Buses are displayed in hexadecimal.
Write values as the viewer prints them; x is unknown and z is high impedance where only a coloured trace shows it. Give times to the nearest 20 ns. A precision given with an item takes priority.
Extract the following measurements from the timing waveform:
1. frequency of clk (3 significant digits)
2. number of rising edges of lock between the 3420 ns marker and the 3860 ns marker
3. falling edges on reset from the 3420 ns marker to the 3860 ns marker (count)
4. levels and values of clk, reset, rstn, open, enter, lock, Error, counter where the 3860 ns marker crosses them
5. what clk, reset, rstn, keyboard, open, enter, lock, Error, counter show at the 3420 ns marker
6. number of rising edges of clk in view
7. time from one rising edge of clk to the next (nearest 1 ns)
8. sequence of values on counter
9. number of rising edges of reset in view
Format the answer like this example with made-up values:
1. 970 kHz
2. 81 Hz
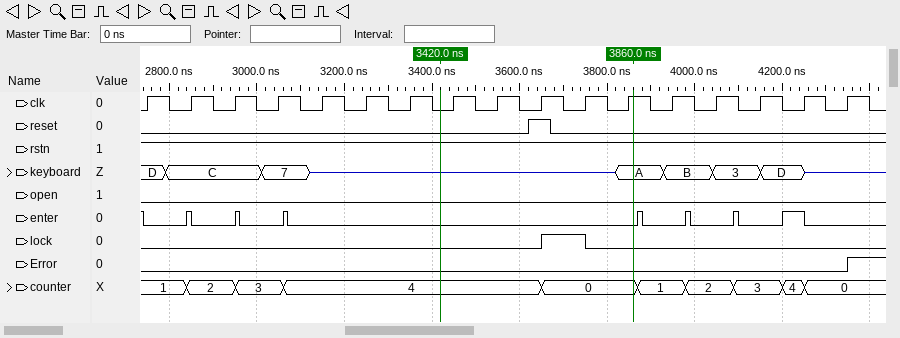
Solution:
1. 10.0 MHz
2. 1
3. 1
4. clk=1, reset=0, rstn=1, open=0, enter=0, lock=0, Error=0, counter=0
5. clk=0, reset=0, rstn=1, keyboard=z, open=0, enter=0, lock=0, Error=0, counter=4
6. 17
7. 100 ns
8. 1, 2, 3, 4, 0, 1, 2, 3, 4, 0
9. 1
